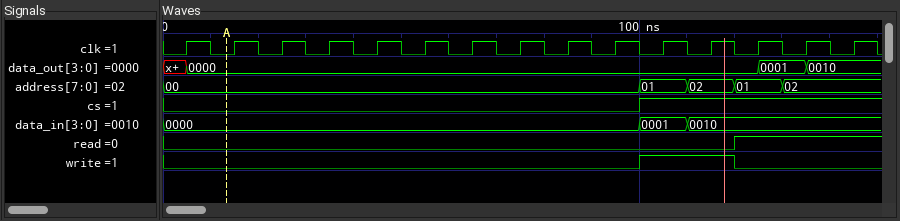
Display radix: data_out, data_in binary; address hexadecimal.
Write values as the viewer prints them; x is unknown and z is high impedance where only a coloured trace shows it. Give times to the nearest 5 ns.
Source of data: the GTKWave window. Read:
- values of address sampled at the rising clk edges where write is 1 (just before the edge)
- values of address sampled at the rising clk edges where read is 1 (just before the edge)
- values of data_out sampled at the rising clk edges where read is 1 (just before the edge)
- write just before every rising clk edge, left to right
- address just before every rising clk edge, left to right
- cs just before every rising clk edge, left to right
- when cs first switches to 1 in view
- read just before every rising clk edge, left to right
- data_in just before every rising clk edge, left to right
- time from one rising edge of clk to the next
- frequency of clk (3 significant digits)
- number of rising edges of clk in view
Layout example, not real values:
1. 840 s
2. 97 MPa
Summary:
1. 01, 02
2. 01, 02, 02
3. 0000, 0001, 0010
4. 0 0 0 0 0 0 0 0 0 0 1 1 0 0 0
5. 00, 00, 00, 00, 00, 00, 00, 00, 00, 00, 01, 02, 01, 02, 02
6. 0 0 0 0 0 0 0 0 0 0 1 1 1 1 1
7. 100 ns
8. 0 0 0 0 0 0 0 0 0 0 0 0 1 1 1
9. 0000, 0000, 0000, 0000, 0000, 0000, 0000, 0000, 0000, 0000, 0001, 0010, 0010, 0010, 0010
10. 10 ns
11. 100 MHz
12. 15
